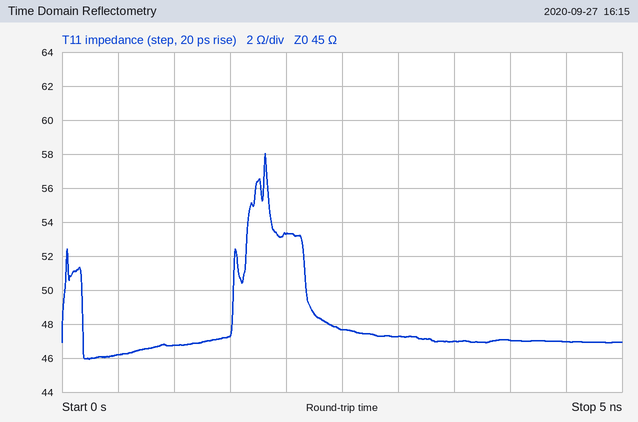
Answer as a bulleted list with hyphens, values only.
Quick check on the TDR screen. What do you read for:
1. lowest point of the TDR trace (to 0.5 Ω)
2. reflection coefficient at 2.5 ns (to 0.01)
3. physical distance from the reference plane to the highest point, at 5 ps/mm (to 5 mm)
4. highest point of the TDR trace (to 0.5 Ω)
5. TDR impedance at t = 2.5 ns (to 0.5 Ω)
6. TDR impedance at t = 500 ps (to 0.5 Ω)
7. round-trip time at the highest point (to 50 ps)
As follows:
- 46.0 Ω
- +0.03
- 180 mm
- 58.0 Ω
- 47.5 Ω
- 46.0 Ω
- 1.80 ns
